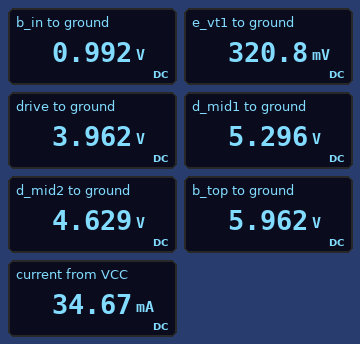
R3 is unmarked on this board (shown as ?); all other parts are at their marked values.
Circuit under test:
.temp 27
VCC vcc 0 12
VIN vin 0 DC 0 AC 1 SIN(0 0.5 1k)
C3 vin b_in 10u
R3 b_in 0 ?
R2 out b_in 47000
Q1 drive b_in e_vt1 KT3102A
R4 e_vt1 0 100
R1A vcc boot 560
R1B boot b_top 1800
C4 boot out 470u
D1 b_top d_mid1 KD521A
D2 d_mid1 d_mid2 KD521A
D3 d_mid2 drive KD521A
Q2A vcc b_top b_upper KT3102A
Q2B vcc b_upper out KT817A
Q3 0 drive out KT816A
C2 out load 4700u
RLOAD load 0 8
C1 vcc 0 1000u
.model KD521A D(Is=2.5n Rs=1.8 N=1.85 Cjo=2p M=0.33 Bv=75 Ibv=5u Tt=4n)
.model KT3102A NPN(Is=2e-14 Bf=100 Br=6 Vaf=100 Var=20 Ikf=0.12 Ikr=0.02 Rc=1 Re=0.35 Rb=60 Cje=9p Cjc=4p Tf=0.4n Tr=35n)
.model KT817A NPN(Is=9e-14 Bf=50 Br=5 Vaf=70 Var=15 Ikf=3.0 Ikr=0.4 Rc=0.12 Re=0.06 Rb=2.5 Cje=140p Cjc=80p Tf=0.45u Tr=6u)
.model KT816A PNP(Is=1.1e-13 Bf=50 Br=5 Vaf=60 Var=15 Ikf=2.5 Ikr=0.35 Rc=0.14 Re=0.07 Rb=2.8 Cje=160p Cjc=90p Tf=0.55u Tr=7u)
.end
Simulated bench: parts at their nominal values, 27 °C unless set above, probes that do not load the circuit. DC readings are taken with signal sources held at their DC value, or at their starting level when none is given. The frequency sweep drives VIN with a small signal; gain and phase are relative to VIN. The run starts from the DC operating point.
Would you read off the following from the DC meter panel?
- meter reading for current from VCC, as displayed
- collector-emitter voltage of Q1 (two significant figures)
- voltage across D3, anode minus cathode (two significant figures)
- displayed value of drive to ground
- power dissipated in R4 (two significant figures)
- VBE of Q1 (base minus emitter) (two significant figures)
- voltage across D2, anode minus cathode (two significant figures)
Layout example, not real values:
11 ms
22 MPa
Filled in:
34.67 mA
3.6 V
670 mV
3.962 V
1.0 mW
670 mV
670 mV
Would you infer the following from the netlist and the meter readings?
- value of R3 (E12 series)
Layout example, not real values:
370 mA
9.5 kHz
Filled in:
22 kΩ
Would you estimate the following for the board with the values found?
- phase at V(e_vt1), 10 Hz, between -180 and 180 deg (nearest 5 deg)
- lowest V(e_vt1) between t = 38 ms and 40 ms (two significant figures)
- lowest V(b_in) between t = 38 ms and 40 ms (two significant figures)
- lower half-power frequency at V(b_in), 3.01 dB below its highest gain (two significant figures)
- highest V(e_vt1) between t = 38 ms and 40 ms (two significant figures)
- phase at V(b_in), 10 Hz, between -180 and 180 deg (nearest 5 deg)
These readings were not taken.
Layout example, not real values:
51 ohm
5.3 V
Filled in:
25 deg
21 mV
620 mV
3.6 Hz
910 mV
25 deg
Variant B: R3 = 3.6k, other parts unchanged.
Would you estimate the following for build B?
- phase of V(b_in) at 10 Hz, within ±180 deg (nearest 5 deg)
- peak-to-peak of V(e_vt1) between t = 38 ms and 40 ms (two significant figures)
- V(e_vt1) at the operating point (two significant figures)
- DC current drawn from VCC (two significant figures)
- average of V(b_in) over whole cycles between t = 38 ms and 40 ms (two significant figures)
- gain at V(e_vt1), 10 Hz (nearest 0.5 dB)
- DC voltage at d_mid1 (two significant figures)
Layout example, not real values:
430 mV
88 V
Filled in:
35 deg
480 mV
52 mV
2.0 mA
660 mV
-5.0 dB
10 V
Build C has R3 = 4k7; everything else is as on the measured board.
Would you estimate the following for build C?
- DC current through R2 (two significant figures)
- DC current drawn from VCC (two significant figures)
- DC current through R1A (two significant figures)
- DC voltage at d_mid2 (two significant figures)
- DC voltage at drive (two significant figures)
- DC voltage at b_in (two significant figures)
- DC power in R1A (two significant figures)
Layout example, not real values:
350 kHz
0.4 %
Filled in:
170 µA
5.7 mA
930 µA
8.6 V
8.0 V
740 mV
480 µW
